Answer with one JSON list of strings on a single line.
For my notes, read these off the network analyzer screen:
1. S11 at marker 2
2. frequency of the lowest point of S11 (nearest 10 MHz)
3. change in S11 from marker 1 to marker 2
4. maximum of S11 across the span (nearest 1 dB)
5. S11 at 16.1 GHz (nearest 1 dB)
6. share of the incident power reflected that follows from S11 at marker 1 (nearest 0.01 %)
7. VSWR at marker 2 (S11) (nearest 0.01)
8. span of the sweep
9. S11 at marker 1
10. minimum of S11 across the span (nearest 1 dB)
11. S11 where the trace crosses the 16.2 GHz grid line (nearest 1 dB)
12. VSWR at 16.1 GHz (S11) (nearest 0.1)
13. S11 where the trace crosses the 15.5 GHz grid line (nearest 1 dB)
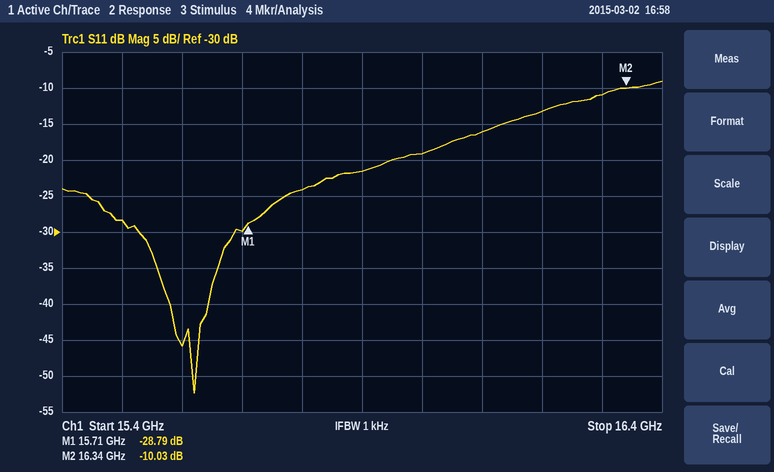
["-10.03 dB", "15.62 GHz", "18.76 dB", "-9 dB", "-16 dB", "0.13 %", "1.92", "1 GHz", "-28.79 dB", "-52 dB", "-13 dB", "1.4", "-28 dB"]
